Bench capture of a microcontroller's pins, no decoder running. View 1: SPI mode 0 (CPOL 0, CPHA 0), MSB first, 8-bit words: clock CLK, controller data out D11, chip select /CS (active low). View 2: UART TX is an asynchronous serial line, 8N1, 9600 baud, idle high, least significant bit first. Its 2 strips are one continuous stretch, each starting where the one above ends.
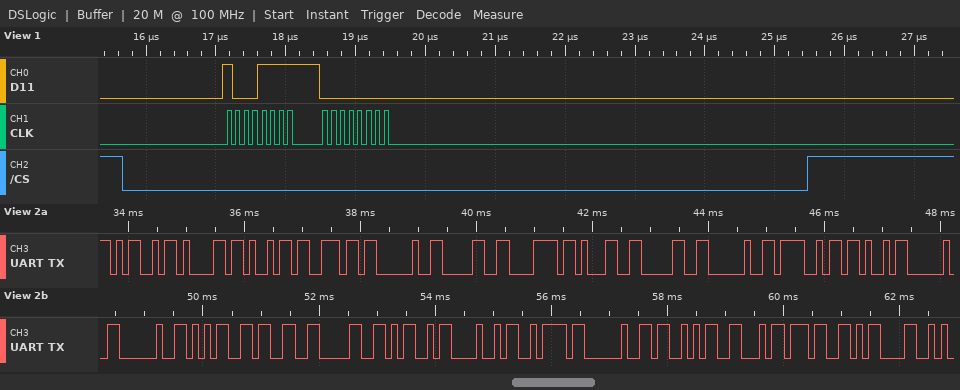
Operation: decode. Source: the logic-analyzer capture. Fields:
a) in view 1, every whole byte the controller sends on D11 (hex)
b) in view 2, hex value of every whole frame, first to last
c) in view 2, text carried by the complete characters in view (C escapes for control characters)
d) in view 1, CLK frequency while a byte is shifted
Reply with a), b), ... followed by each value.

a) 8F 00
b) 4D 61 69 6E 20 30 78 31 30 20 4F 4B 20 20 35 33 30 4D 48 7A 20 53 46 37 0D
c) "Main 0x10 OK  530MHz SF7\r"
d) 8 MHz
